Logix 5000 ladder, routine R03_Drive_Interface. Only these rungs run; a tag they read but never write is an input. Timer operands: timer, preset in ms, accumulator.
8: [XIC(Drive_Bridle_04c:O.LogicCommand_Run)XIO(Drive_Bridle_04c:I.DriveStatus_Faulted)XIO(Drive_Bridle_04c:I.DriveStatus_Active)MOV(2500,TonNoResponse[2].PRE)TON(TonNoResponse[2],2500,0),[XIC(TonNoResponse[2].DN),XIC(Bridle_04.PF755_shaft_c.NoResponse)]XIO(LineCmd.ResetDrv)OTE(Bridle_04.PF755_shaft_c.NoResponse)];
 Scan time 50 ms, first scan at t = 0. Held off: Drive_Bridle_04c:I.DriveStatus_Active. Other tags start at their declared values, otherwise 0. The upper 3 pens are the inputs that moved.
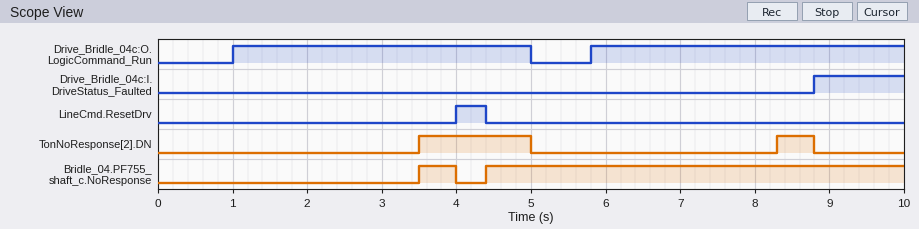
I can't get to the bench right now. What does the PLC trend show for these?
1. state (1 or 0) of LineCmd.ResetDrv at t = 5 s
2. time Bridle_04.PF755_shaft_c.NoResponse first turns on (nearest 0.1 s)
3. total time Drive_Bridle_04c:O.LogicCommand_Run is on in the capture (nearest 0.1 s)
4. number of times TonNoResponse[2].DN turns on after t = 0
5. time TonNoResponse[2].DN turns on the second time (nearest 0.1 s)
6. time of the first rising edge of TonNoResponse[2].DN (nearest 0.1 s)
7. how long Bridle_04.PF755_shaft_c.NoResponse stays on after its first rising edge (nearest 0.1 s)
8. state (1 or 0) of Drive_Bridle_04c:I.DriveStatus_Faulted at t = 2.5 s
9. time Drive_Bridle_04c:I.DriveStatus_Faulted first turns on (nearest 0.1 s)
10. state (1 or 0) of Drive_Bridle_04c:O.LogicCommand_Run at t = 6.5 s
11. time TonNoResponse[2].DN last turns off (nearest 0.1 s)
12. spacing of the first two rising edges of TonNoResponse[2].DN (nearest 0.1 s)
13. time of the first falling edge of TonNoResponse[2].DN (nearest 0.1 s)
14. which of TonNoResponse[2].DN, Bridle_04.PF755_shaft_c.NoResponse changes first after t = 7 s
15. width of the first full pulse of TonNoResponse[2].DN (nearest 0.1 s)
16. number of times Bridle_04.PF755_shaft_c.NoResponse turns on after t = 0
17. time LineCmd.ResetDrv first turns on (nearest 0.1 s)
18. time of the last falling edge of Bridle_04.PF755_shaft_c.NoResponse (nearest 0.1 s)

0
3.5 s
8.2 s
2
8.3 s
3.5 s
0.5 s
0
8.8 s
1
8.8 s
4.8 s
5.0 s
TonNoResponse[2].DN
1.5 s
2
4.0 s
4.0 s
